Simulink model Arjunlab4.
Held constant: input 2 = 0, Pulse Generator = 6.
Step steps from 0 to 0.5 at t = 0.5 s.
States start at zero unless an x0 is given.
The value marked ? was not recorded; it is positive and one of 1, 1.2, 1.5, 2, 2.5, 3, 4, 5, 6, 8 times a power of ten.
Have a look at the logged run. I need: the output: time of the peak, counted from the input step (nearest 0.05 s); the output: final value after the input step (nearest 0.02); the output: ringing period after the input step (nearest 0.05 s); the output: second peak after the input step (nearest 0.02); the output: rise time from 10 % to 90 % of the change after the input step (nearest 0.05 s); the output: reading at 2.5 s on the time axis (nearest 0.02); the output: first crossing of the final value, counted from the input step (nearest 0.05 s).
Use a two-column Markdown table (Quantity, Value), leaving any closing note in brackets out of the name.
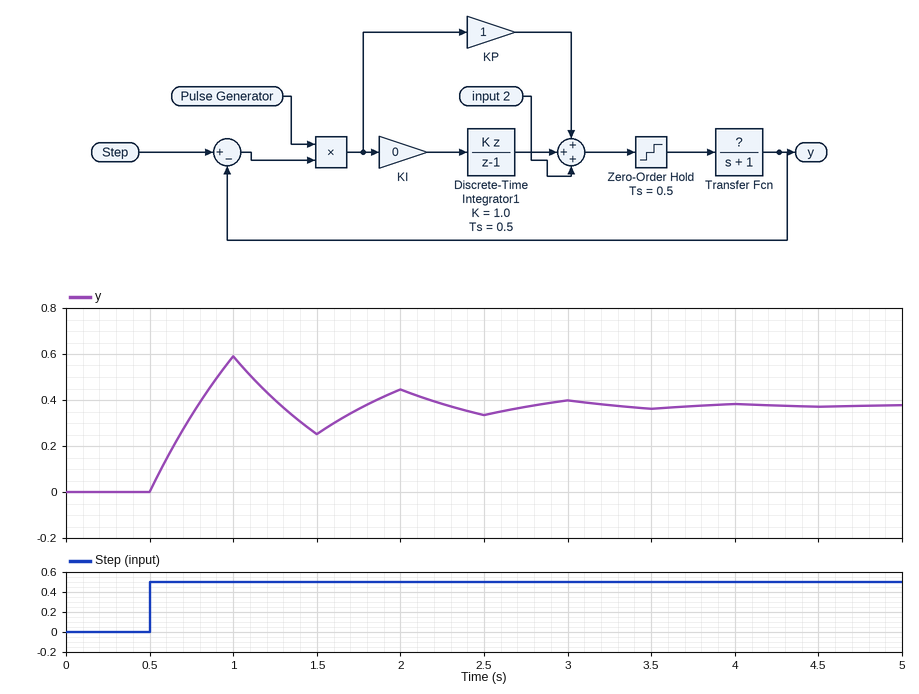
| Quantity | Value |
|---|---|
| the output: time of the peak, counted from the input step | 0.50 s |
| the output: final value after the input step | 0.38 |
| the output: ringing period after the input step | 1.00 s |
| the output: second peak after the input step | 0.44 |
| the output: rise time from 10 % to 90 % of the change after the input step | 0.25 s |
| the output: reading at 2.5 s on the time axis | 0.34 |
| the output: first crossing of the final value, counted from the input step | 0.30 s |
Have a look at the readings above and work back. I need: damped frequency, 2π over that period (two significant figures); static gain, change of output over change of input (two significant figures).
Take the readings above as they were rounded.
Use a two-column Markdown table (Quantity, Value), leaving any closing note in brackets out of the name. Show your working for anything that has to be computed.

| Quantity | Value |
|---|---|
| damped frequency, 2π over that period | 2π / 1 = 6.3 rad/s |
| static gain, change of output over change of input | (0.38 - 0) / (0.5 - 0) = 0.76 |
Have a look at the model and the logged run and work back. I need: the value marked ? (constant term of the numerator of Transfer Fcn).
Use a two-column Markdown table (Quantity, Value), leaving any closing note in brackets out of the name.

| Quantity | Value |
|---|---|
| the value marked ? | 0.5 |
